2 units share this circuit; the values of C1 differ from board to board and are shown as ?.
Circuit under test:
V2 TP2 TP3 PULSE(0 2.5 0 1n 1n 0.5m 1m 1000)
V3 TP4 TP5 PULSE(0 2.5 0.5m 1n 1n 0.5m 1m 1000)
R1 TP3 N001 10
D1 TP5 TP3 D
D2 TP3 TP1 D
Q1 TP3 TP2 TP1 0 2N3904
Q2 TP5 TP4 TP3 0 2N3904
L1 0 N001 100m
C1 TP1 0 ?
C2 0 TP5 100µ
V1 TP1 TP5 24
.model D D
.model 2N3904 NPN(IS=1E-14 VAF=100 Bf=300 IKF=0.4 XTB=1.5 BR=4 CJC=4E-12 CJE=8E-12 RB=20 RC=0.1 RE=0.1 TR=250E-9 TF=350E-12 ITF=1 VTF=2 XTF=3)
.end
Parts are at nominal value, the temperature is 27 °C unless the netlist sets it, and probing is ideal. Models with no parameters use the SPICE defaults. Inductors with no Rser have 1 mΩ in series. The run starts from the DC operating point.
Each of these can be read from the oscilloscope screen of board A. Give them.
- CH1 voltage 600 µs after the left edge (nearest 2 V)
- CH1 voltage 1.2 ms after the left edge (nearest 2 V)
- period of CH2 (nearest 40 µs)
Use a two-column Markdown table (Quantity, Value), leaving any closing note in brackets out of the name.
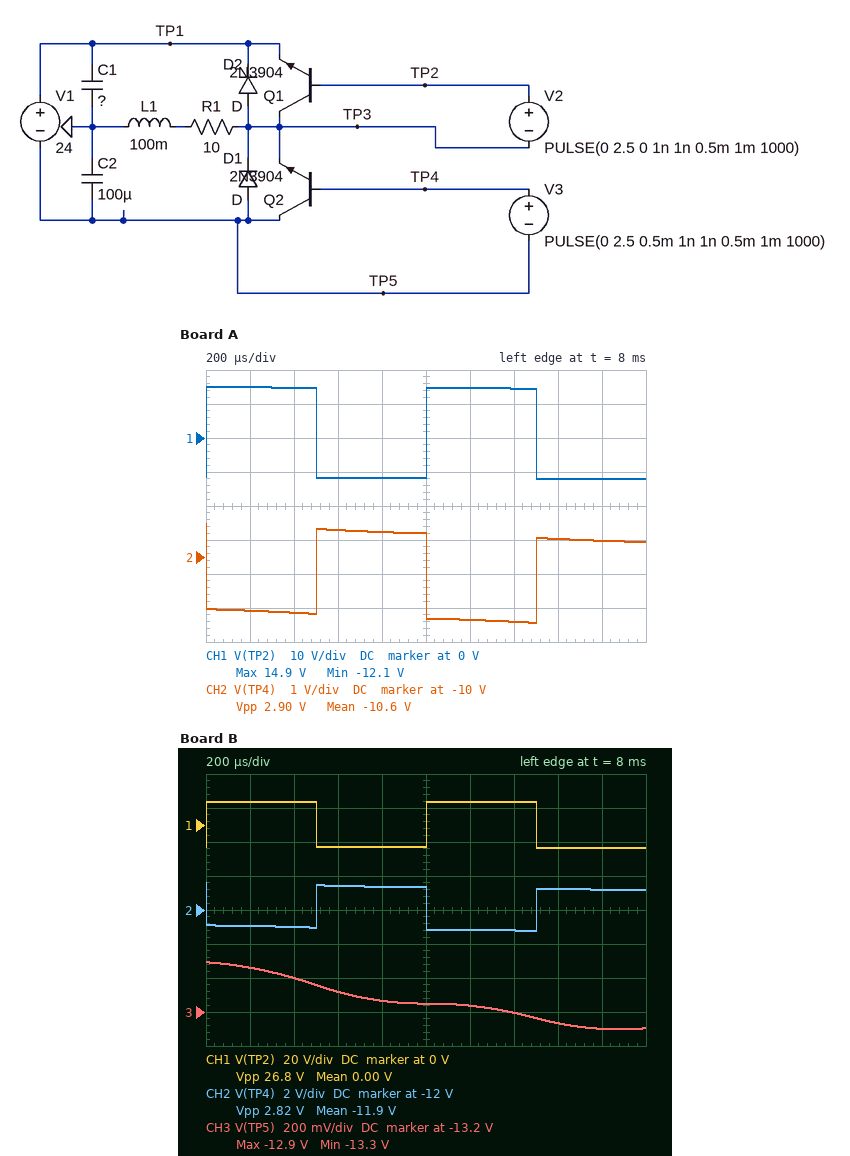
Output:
| Quantity | Value |
|---|---|
| CH1 voltage 600 µs after the left edge | -12 V |
| CH1 voltage 1.2 ms after the left edge | 14 V |
| period of CH2 | 1.00 ms |
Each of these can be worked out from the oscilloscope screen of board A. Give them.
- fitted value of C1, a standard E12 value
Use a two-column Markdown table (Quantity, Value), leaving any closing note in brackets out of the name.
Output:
| Quantity | Value |
|---|---|
| fitted value of C1, a standard E12 value | 220 µF |
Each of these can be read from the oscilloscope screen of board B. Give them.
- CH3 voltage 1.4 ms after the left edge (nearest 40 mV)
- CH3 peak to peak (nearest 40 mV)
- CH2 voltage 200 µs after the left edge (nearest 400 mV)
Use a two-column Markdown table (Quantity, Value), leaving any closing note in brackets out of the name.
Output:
| Quantity | Value |
|---|---|
| CH3 voltage 1.4 ms after the left edge | -13.20 V |
| CH3 peak to peak | 400 mV |
| CH2 voltage 200 µs after the left edge | -12.8 V |
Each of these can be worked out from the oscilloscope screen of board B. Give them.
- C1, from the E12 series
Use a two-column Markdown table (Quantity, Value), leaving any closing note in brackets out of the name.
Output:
| Quantity | Value |
|---|---|
| C1, from the E12 series | 47 µF |
